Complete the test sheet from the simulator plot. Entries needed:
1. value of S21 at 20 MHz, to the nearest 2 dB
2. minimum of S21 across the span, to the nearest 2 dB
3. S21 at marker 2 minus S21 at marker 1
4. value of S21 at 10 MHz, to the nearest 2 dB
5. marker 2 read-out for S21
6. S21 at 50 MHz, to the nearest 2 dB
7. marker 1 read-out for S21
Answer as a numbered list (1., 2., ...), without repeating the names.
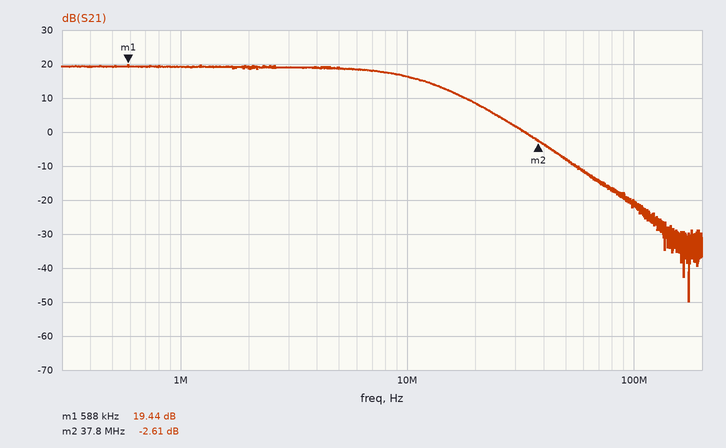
1. 8 dB
2. -50 dB
3. -22.05 dB
4. 16 dB
5. -2.61 dB
6. -8 dB
7. 19.44 dB
